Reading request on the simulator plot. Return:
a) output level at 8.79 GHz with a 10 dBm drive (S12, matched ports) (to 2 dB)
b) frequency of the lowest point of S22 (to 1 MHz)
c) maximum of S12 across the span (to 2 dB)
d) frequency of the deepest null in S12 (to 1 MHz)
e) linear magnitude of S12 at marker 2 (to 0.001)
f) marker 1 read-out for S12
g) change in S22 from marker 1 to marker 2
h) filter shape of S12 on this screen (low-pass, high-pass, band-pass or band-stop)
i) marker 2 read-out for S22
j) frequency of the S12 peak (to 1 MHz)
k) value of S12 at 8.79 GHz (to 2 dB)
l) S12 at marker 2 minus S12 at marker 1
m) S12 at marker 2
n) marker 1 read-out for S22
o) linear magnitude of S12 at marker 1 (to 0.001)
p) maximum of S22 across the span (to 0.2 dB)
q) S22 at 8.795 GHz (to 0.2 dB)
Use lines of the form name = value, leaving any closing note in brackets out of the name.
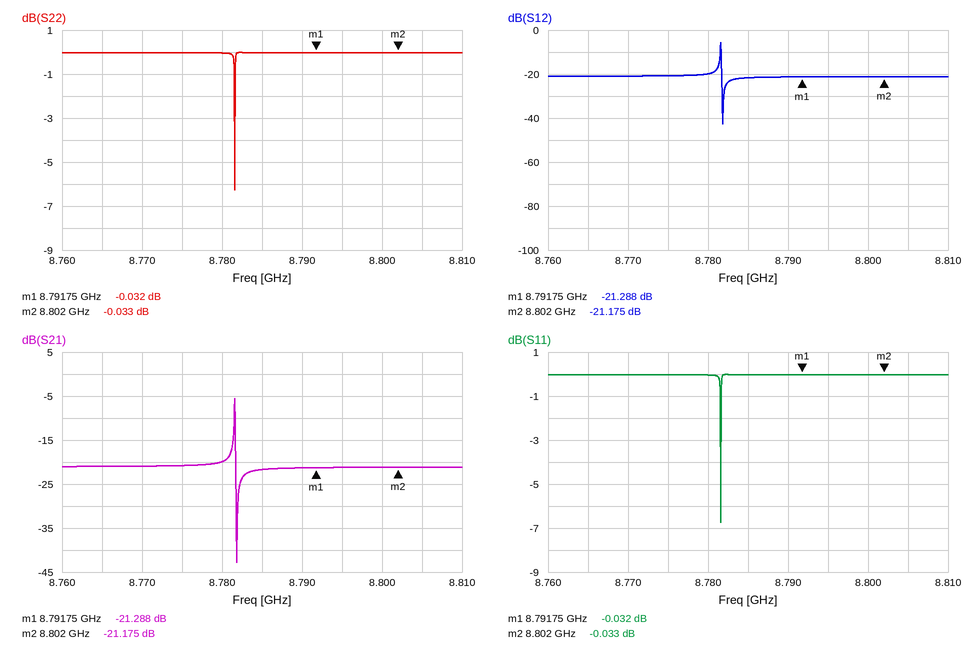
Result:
output level at 8.79 GHz with a 10 dBm drive (S12, matched ports) = -12 dBm
frequency of the lowest point of S22 = 8.782 GHz
maximum of S12 across the span = -6 dB
frequency of the deepest null in S12 = 8.782 GHz
linear magnitude of S12 at marker 2 = 0.087
marker 1 read-out for S12 = -21.288 dB
change in S22 from marker 1 to marker 2 = -0.001 dB
filter shape of S12 on this screen = band-pass
marker 2 read-out for S22 = -0.033 dB
frequency of the S12 peak = 8.782 GHz
value of S12 at 8.79 GHz = -22 dB
S12 at marker 2 minus S12 at marker 1 = 0.113 dB
S12 at marker 2 = -21.175 dB
marker 1 read-out for S22 = -0.032 dB
linear magnitude of S12 at marker 1 = 0.086
maximum of S22 across the span = 0.0 dB
S22 at 8.795 GHz = 0.0 dB
